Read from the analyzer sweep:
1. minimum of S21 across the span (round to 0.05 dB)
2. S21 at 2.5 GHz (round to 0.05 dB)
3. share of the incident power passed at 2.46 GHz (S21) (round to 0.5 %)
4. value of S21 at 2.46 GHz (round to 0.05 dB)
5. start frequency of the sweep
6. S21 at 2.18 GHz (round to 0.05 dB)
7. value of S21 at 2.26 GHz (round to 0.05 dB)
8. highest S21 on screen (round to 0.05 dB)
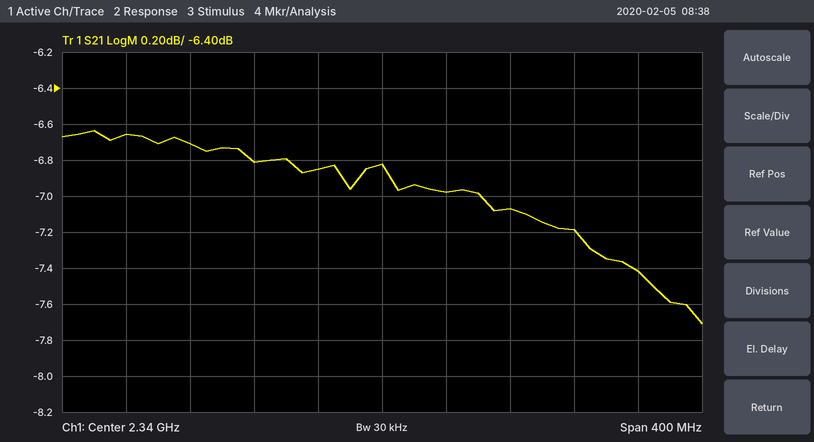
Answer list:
-7.70 dB
-7.40 dB
19.0 %
-7.20 dB
2.14 GHz
-6.65 dB
-6.80 dB
-6.65 dB
